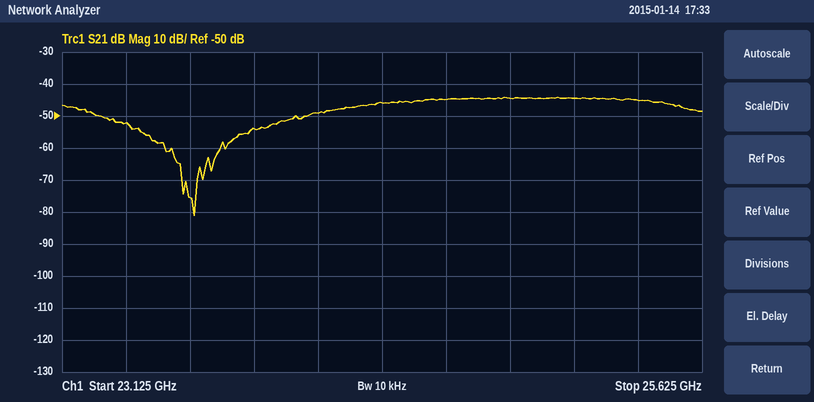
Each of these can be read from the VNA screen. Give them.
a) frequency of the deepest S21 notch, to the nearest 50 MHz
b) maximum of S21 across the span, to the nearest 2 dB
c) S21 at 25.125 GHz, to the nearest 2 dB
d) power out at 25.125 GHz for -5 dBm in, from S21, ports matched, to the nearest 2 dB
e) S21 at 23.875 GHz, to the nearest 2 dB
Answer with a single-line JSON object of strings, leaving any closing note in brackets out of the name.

{"frequency of the deepest S21 notch, to the nearest 50 MHz": "23.65 GHz", "maximum of S21 across the span, to the nearest 2 dB": "-44 dB", "S21 at 25.125 GHz, to the nearest 2 dB": "-44 dB", "power out at 25.125 GHz for -5 dBm in, from S21, ports matched, to the nearest 2 dB": "-50 dBm", "S21 at 23.875 GHz, to the nearest 2 dB": "-54 dB"}
